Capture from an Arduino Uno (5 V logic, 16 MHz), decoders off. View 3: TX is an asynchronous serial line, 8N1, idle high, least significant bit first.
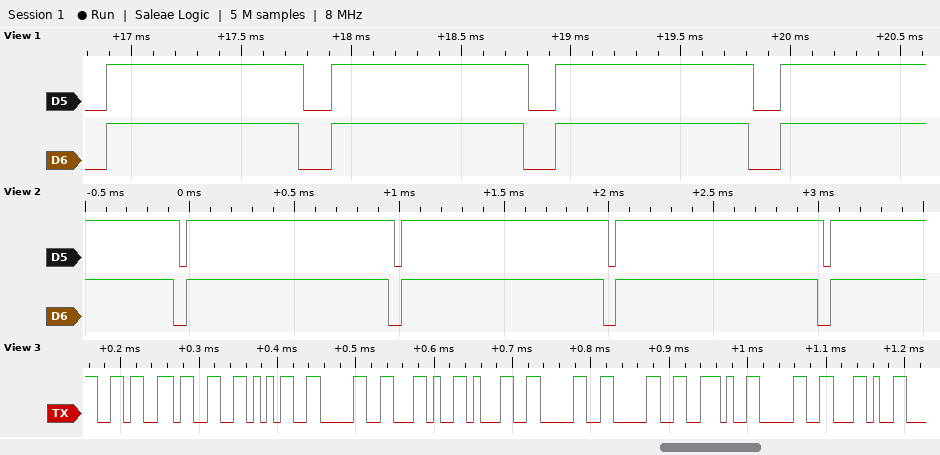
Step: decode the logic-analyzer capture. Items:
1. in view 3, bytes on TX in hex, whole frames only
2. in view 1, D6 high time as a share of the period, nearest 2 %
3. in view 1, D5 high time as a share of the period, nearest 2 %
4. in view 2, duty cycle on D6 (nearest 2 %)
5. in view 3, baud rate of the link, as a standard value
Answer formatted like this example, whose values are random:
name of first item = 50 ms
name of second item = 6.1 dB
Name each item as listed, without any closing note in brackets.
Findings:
in view 3, bytes on TX in hex, whole frames only = 0x36 0x33 0x35 0x30 0x2C 0x31 0x30 0x30 0x2E 0x30 0x2C
in view 1, D6 high time as a share of the period, nearest 2 % = 86 %
in view 1, D5 high time as a share of the period, nearest 2 % = 88 %
in view 2, duty cycle on D6 = 94 %
in view 3, baud rate of the link, as a standard value = 115200 baud
